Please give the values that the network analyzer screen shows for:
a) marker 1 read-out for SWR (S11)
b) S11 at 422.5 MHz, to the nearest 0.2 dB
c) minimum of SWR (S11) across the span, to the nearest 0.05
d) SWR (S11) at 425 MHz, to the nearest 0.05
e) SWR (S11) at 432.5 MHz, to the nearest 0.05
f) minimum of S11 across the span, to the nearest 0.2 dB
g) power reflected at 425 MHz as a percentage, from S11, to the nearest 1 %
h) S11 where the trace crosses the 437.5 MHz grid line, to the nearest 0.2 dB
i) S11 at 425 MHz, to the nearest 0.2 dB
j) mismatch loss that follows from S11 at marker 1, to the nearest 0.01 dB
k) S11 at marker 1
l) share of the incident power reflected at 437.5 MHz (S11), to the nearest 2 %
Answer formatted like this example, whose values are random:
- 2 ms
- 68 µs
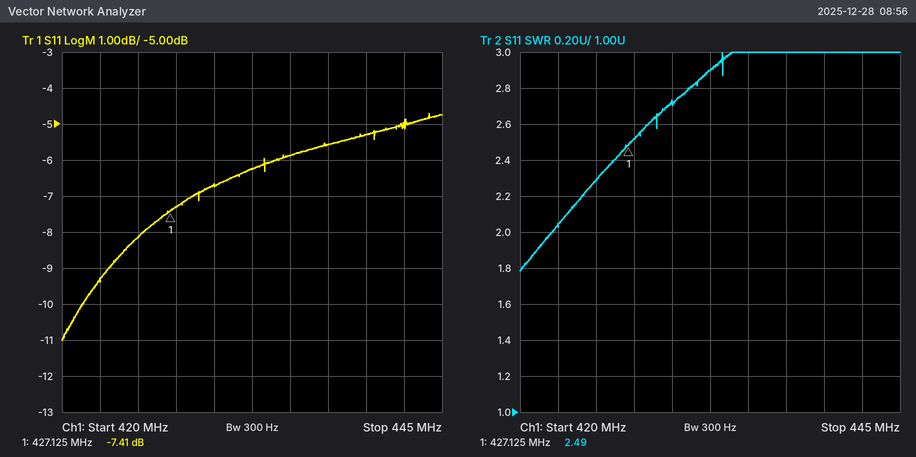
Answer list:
- 2.49
- -9.4 dB
- 1.80
- 2.30
- 2.90
- -11.0 dB
- 15 %
- -5.6 dB
- -8.2 dB
- 0.87 dB
- -7.41 dB
- 28 %
